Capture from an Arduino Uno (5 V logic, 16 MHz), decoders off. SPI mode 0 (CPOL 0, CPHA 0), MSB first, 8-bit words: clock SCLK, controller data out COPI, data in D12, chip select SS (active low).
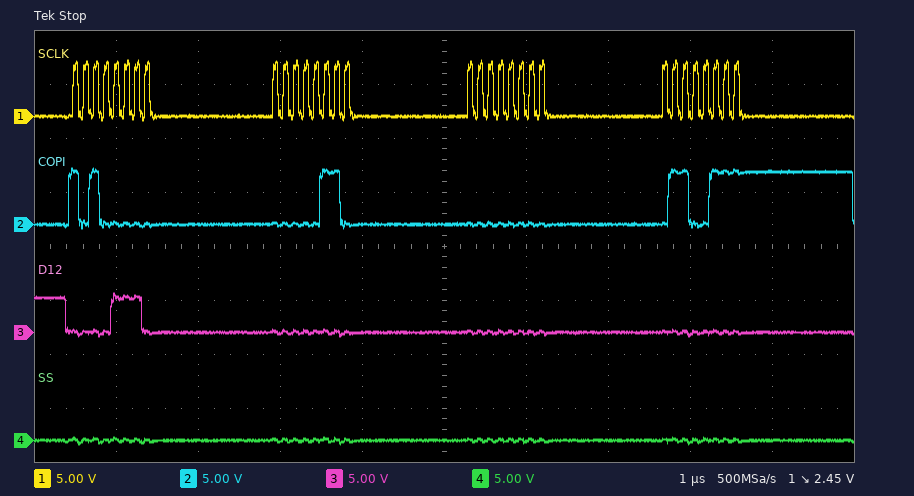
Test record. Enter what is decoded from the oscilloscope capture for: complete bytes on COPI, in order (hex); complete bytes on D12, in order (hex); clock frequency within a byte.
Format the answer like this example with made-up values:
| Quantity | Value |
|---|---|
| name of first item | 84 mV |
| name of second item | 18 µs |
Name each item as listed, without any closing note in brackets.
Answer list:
| Quantity | Value |
|---|---|
| complete bytes on COPI, in order | A0 06 00 67 |
| complete bytes on D12, in order | 0E 00 00 00 |
| clock frequency within a byte | 8 MHz |
